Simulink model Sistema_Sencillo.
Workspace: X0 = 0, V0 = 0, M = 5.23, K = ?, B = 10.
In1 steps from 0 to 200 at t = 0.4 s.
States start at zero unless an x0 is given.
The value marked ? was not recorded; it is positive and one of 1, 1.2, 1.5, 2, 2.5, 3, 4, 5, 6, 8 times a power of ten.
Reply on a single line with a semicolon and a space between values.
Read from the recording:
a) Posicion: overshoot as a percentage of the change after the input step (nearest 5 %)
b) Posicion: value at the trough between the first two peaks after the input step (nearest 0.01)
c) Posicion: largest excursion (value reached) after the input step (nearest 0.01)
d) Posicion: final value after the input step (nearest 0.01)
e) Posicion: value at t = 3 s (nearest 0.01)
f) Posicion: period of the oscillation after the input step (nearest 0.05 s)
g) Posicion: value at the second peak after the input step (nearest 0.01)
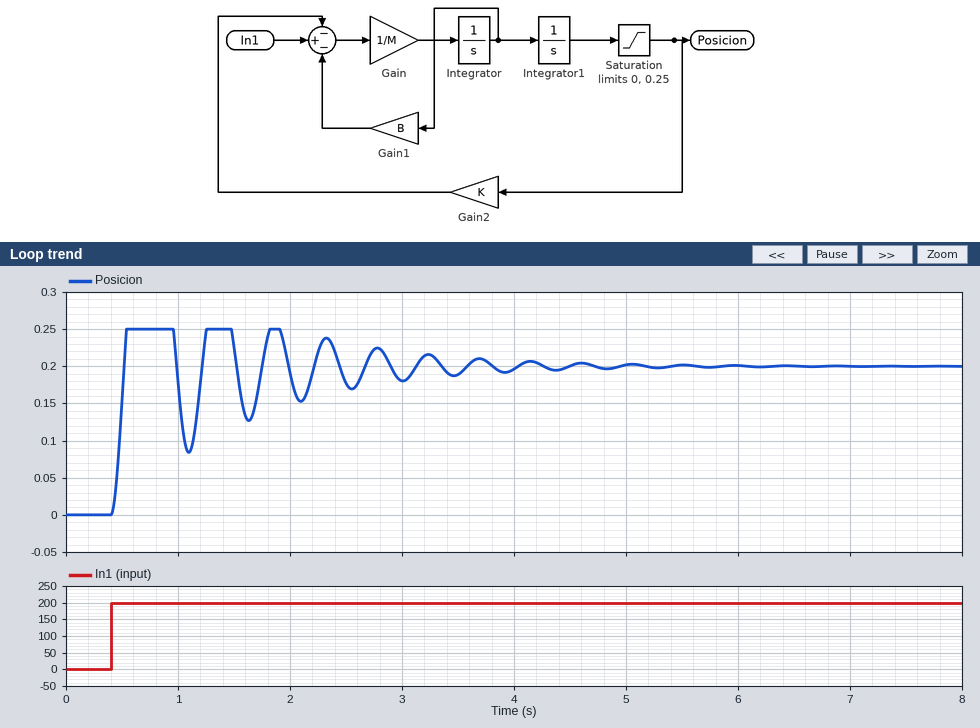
25 %; 0.08; 0.25; 0.20; 0.18; 0.60 s; 0.25
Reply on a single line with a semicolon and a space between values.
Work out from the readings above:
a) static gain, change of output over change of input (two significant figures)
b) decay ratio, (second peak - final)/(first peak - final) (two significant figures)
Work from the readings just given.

0.0010; 1.0
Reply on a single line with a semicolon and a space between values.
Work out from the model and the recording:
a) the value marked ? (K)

1000
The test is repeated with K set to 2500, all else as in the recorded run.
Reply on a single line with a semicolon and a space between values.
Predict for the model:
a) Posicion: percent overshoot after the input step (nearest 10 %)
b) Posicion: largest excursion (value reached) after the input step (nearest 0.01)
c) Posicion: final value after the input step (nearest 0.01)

90 %; 0.15; 0.08
